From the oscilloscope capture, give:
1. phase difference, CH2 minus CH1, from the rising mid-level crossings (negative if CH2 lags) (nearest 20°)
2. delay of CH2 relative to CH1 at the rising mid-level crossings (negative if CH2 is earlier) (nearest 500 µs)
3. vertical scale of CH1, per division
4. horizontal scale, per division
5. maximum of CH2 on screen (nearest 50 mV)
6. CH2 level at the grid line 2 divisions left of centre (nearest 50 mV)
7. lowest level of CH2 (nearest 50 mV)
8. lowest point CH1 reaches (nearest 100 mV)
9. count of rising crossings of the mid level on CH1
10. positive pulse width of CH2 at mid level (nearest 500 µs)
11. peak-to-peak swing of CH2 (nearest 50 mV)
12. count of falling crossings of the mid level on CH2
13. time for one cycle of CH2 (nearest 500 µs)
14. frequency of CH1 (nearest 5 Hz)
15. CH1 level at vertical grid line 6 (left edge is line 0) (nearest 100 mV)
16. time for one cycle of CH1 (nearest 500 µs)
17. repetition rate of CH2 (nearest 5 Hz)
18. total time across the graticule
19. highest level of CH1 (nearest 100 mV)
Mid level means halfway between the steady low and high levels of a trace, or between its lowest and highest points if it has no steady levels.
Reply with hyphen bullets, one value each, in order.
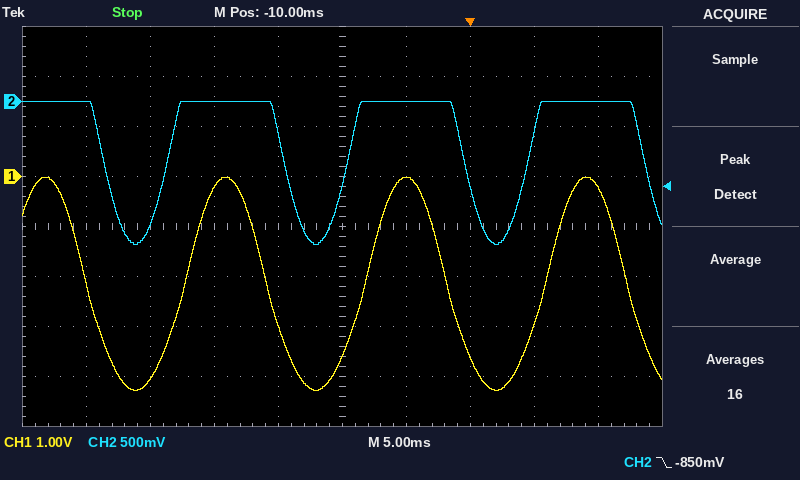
- +40°
- -1.5 ms
- 1 V
- 5 ms
- 0 mV
- 0 mV
- -1.45 V
- -4.3 V
- 3
- 9.5 ms
- 1.45 V
- 4
- 14.0 ms
- 70 Hz
- 0.0 V
- 14.0 ms
- 70 Hz
- 50 ms
- 0.0 V
